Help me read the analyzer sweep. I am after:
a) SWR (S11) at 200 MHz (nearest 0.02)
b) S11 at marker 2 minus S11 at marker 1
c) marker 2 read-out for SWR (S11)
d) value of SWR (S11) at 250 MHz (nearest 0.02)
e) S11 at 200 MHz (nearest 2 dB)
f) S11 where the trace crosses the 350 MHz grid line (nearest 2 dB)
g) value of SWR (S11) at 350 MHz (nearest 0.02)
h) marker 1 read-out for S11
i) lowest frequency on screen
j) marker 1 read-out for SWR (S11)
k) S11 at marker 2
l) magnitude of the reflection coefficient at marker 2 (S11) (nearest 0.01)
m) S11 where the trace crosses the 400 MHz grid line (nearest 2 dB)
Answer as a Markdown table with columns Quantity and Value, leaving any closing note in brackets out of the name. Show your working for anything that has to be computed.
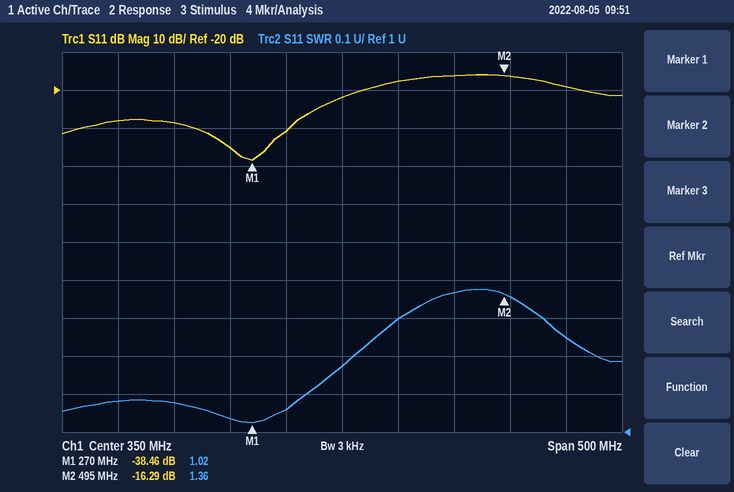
| Quantity | Value |
|---|---|
| SWR (S11) at 200 MHz | 1.08 |
| S11 at marker 2 minus S11 at marker 1 | -16.29 − (-38.46) = 22.17 dB |
| marker 2 read-out for SWR | 1.36 |
| value of SWR (S11) at 250 MHz | 1.04 |
| S11 at 200 MHz | -28 dB |
| S11 where the trace crosses the 350 MHz grid line | -22 dB |
| value of SWR (S11) at 350 MHz | 1.18 |
| marker 1 read-out for S11 | -38.46 dB |
| lowest frequency on screen | 100 MHz |
| marker 1 read-out for SWR | 1.02 |
| S11 at marker 2 | -16.29 dB |
| magnitude of the reflection coefficient at marker 2 (S11) | 10^(-16.29/20) ≈ 0.15 |
| S11 where the trace crosses the 400 MHz grid line | -18 dB |
